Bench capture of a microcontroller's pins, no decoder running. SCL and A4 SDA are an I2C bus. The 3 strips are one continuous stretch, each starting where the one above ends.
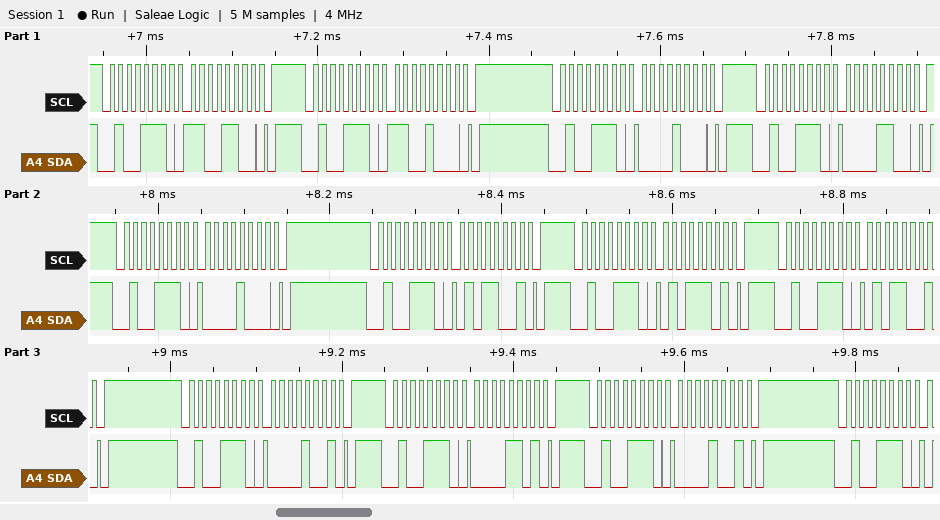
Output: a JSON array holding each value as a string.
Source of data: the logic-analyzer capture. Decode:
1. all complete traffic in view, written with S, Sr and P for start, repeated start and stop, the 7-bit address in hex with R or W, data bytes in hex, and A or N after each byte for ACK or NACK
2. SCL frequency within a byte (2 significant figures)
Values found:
["S 27W A CC A P S 27W A C8 A P S 27W A 08 A P S 27W A 0C A P S 27W A 08 A P S 27W A 59 A P S 27W A 5D A P S 27W A 59 A P S 27W A 09 A P S 27W A 0D A P S 27W A 09 A P S 27W A", "100 kHz"]
